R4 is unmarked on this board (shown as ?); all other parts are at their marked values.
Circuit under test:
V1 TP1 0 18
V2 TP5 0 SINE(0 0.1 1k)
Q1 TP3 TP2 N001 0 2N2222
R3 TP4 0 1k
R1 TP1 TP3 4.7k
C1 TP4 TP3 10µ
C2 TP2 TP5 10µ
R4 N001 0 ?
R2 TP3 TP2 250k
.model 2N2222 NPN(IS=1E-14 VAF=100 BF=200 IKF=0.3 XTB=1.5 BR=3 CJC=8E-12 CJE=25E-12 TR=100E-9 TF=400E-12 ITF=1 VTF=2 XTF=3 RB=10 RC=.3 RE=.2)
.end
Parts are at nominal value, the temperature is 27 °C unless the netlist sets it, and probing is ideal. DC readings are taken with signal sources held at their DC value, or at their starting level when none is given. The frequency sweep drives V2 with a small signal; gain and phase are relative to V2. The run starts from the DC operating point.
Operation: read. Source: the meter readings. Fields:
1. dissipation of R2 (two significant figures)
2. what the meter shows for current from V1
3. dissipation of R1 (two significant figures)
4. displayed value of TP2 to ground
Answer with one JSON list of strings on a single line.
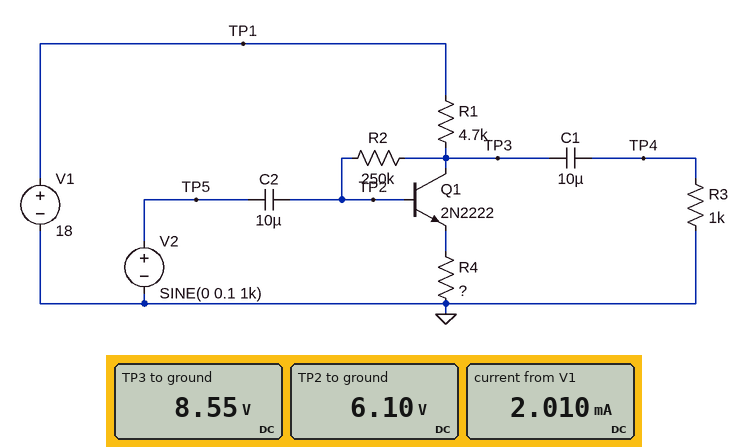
["24 µW", "2.010 mA", "19 mW", "6.10 V"]
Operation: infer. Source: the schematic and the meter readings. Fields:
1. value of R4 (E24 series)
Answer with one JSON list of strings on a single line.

["2.7 kΩ"]
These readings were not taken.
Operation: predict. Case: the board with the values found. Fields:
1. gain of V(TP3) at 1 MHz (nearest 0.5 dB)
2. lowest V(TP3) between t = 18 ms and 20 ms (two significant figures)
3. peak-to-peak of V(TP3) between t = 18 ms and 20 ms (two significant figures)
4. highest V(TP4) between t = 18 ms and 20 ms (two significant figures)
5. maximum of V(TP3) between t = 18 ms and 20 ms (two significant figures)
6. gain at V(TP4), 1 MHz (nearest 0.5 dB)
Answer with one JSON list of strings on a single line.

["-10.5 dB", "8.5 V", "60 mV", "30 mV", "8.6 V", "-10.5 dB"]
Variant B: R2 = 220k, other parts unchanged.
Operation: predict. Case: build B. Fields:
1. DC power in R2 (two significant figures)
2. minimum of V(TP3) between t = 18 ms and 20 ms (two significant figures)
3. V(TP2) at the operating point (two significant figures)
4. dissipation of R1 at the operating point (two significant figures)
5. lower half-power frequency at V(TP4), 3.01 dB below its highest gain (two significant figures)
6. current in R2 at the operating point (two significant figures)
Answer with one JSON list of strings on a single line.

["22 µW", "8.4 V", "6.2 V", "20 mW", "31 MHz", "10 µA"]
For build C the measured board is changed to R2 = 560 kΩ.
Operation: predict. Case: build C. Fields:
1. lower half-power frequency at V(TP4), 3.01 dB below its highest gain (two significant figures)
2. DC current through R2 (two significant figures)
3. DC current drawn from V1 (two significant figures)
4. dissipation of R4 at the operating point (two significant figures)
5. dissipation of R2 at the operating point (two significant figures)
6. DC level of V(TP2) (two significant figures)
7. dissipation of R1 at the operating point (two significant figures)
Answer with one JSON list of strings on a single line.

["36 MHz", "8.2 µA", "1.7 mA", "8.0 mW", "38 µW", "5.3 V", "14 mW"]
